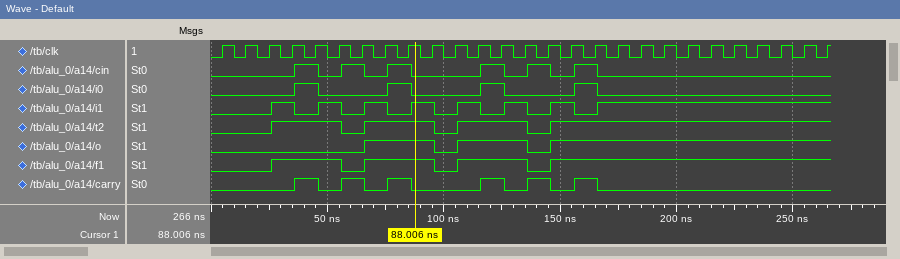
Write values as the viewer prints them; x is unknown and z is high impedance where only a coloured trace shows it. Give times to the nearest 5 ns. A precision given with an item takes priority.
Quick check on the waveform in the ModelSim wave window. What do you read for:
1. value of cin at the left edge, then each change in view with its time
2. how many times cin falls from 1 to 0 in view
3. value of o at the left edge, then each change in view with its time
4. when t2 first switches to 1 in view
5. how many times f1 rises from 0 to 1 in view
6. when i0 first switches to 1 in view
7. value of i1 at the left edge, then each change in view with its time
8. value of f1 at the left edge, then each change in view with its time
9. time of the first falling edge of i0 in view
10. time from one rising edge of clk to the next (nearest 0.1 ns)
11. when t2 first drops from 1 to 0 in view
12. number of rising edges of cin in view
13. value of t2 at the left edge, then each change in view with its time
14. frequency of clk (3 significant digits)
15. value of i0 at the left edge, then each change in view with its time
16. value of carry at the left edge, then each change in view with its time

0, 1 at 35 ns, 0 at 45 ns, 1 at 55 ns, 0 at 65 ns, 1 at 75 ns, 0 at 85 ns, 1 at 115 ns, 0 at 125 ns, 1 at 135 ns, 0 at 145 ns, 1 at 155 ns, 0 at 165 ns
6
0, 1 at 65 ns, 0 at 95 ns, 1 at 105 ns, 0 at 135 ns, 1 at 145 ns
25 ns
4
35 ns
0, 1 at 25 ns, 0 at 35 ns, 1 at 45 ns, 0 at 55 ns, 1 at 65 ns, 0 at 75 ns, 1 at 85 ns, 0 at 95 ns, 1 at 105 ns, 0 at 115 ns, 1 at 125 ns, 0 at 135 ns, 1 at 145 ns, 0 at 155 ns, 1 at 165 ns
0, 1 at 25 ns, 0 at 55 ns, 1 at 65 ns, 0 at 95 ns, 1 at 105 ns, 0 at 135 ns, 1 at 145 ns
45 ns
10 ns
55 ns
6
0, 1 at 25 ns, 0 at 55 ns, 1 at 65 ns, 0 at 95 ns, 1 at 105 ns, 0 at 135 ns, 1 at 145 ns
100 MHz
0, 1 at 35 ns, 0 at 45 ns, 1 at 75 ns, 0 at 85 ns, 1 at 115 ns, 0 at 125 ns, 1 at 155 ns, 0 at 165 ns
0, 1 at 35 ns, 0 at 45 ns, 1 at 55 ns, 0 at 65 ns, 1 at 75 ns, 0 at 85 ns, 1 at 115 ns, 0 at 125 ns, 1 at 135 ns, 0 at 145 ns, 1 at 155 ns, 0 at 165 ns
